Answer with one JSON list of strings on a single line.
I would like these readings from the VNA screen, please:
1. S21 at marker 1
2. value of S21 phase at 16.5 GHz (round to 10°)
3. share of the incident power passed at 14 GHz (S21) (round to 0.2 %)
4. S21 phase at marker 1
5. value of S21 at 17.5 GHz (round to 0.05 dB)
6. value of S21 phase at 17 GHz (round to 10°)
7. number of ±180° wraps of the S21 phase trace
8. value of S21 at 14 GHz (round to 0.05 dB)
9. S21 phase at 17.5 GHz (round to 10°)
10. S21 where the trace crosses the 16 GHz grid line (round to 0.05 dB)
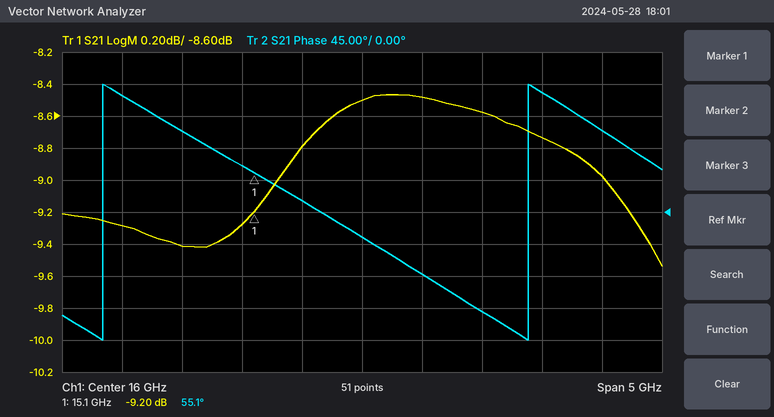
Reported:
["-9.20 dB", "-90°", "11.8 %", "55.1°", "-8.75 dB", "-140°", "2", "-9.30 dB", "170°", "-8.50 dB"]
